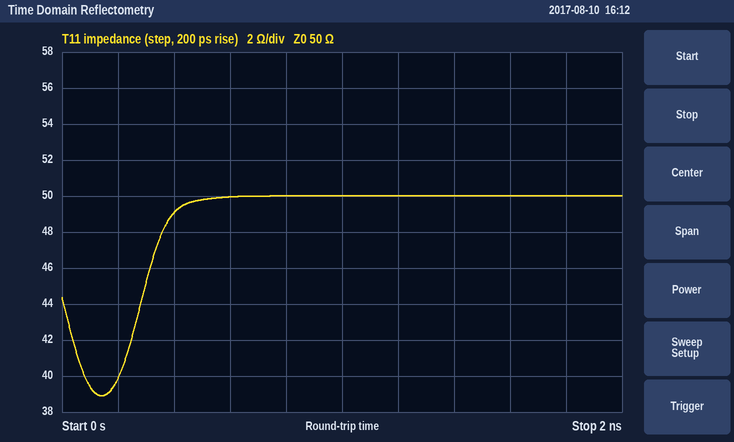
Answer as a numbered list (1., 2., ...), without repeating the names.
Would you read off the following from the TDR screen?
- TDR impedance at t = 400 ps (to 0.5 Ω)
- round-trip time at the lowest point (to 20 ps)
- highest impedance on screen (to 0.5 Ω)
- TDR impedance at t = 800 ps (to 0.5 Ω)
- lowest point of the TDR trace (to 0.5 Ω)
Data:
1. 49.0 Ω
2. 140 ps
3. 50.0 Ω
4. 50.0 Ω
5. 39.0 Ω
